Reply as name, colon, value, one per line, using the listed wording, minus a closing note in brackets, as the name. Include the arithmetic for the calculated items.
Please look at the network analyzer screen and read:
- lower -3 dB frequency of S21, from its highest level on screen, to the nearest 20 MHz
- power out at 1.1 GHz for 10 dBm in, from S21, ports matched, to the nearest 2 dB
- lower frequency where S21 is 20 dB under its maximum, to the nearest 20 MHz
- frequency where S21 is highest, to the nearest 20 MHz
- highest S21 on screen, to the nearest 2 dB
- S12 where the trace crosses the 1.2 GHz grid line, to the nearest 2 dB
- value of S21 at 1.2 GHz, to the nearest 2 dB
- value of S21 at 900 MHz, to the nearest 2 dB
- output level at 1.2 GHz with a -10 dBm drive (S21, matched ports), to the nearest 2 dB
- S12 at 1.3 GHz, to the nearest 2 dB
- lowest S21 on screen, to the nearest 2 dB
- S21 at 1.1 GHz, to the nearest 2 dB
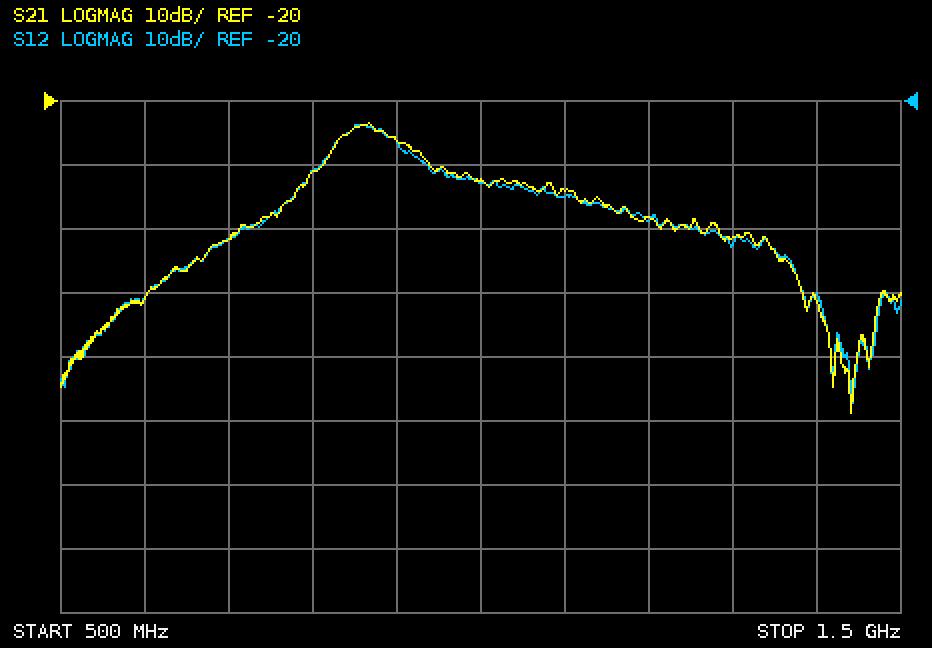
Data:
lower -3 dB frequency of S21, from its highest level on screen, to the nearest 20 MHz: 820 MHz
power out at 1.1 GHz for 10 dBm in, from S21, ports matched, to the nearest 2 dB: 10 dBm + (-34 dB) = -24 dBm
lower frequency where S21 is 20 dB under its maximum, to the nearest 20 MHz: 680 MHz
frequency where S21 is highest, to the nearest 20 MHz: 860 MHz
highest S21 on screen, to the nearest 2 dB: -24 dB
S12 where the trace crosses the 1.2 GHz grid line, to the nearest 2 dB: -38 dB
value of S21 at 1.2 GHz, to the nearest 2 dB: -38 dB
value of S21 at 900 MHz, to the nearest 2 dB: -26 dB
output level at 1.2 GHz with a -10 dBm drive (S21, matched ports), to the nearest 2 dB: -10 dBm + (-38 dB) = -48 dBm
S12 at 1.3 GHz, to the nearest 2 dB: -42 dB
lowest S21 on screen, to the nearest 2 dB: -68 dB
S21 at 1.1 GHz, to the nearest 2 dB: -34 dB
